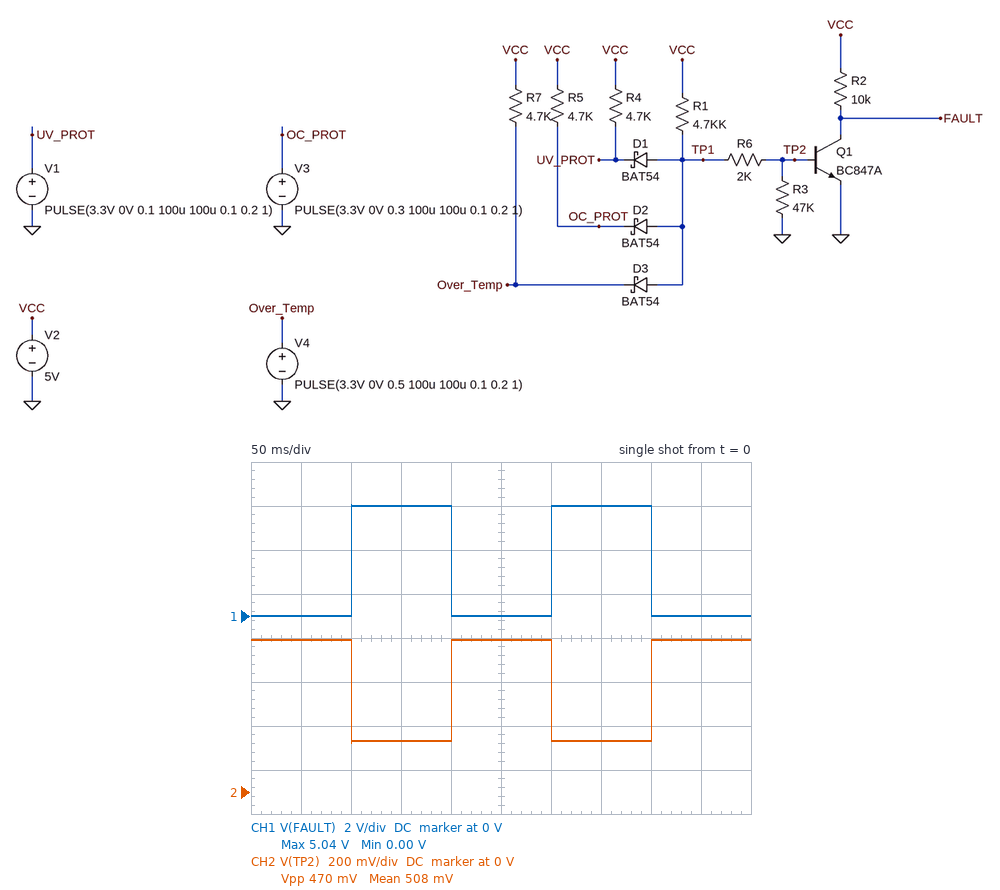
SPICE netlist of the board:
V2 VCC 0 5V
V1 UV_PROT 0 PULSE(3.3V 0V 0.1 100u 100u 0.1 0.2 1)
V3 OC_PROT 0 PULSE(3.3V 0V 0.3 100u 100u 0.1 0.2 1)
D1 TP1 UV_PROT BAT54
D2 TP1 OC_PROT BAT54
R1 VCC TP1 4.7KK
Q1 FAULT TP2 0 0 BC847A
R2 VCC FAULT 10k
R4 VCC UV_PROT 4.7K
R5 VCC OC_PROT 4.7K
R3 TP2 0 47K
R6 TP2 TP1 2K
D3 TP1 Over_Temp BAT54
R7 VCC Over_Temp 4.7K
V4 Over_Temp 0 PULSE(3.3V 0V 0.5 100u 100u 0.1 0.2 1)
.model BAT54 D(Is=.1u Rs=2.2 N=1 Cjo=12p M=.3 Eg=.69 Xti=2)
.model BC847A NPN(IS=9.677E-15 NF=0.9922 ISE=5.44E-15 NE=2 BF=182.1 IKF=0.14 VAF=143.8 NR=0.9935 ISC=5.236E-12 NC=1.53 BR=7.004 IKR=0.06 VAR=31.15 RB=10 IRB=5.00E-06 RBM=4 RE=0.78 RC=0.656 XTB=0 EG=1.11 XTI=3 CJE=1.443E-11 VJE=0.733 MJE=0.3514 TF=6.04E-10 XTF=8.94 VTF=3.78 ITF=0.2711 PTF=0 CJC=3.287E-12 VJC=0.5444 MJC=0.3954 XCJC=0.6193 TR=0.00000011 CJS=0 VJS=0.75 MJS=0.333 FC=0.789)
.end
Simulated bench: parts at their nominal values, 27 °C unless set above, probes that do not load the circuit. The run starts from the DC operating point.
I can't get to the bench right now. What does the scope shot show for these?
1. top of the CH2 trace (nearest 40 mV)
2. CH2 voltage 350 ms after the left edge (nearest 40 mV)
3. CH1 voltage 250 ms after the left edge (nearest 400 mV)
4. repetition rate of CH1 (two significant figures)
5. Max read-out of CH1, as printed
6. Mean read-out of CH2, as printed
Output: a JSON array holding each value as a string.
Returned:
["680 mV", "240 mV", "0 V", "5.0 Hz", "5.04 V", "508 mV"]
